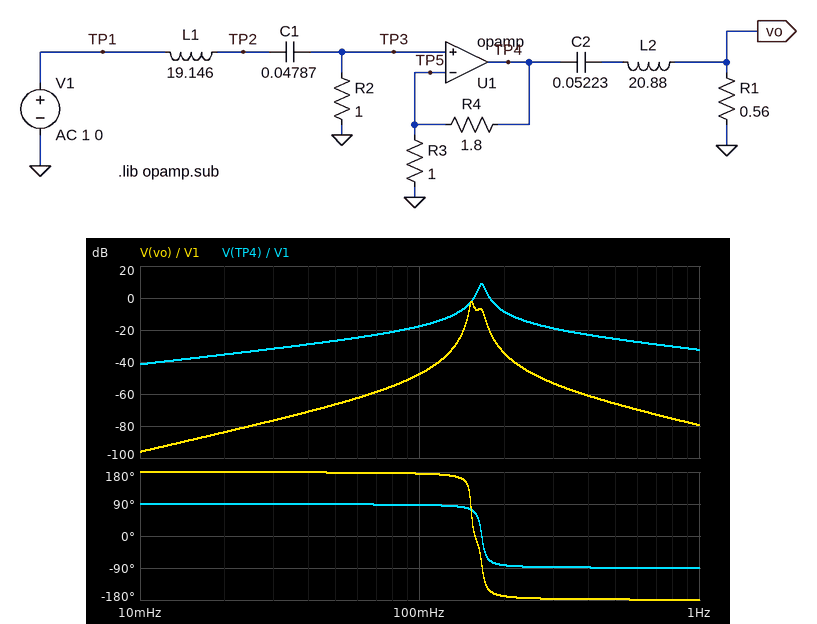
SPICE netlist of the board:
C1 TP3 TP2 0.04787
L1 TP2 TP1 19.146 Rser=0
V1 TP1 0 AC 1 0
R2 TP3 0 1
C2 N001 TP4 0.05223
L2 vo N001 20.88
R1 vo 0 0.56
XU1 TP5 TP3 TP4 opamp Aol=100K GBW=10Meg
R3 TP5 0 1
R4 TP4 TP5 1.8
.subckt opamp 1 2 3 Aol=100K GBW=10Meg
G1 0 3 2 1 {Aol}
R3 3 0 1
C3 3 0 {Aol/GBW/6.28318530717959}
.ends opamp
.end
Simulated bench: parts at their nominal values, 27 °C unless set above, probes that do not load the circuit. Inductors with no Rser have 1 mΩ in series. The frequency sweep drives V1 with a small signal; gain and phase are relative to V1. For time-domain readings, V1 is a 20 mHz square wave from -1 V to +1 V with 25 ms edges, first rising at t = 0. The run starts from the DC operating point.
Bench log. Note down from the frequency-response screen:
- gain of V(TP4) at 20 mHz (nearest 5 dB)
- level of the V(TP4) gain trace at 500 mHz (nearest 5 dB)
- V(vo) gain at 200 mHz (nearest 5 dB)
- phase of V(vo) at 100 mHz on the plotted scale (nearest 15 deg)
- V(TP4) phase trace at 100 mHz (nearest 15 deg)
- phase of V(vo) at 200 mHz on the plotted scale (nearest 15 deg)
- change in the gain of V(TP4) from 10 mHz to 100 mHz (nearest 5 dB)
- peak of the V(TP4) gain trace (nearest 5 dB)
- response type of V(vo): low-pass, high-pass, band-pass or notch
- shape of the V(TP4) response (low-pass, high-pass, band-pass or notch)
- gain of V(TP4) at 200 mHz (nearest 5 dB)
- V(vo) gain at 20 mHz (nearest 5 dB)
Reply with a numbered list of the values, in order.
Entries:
1. -35 dB
2. -25 dB
3. -35 dB
4. 180 deg
5. 90 deg
6. -165 deg
7. 25 dB
8. 10 dB
9. band-pass
10. band-pass
11. -10 dB
12. -85 dB
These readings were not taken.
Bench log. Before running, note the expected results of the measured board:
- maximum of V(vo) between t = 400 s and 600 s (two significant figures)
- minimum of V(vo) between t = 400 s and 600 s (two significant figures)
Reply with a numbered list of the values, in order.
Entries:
1. 24 mV
2. -24 mV
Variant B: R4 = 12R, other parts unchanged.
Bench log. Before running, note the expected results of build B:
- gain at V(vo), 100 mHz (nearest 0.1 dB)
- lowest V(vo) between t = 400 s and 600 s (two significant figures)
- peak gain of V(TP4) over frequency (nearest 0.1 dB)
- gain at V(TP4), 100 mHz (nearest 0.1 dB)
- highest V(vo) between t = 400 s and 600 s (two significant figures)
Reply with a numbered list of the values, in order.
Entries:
1. -34.1 dB
2. -110 mV
3. 22.3 dB
4. -4.3 dB
5. 110 mV
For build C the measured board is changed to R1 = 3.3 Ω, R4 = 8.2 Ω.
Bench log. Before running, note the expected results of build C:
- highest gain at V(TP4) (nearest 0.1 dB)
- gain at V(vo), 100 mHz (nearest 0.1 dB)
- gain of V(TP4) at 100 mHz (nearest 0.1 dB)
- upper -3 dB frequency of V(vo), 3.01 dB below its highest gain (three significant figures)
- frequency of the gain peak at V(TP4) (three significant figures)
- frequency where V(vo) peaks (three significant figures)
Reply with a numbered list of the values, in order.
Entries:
1. 19.3 dB
2. -21.8 dB
3. -7.3 dB
4. 169 mHz
5. 166 mHz
6. 166 mHz
